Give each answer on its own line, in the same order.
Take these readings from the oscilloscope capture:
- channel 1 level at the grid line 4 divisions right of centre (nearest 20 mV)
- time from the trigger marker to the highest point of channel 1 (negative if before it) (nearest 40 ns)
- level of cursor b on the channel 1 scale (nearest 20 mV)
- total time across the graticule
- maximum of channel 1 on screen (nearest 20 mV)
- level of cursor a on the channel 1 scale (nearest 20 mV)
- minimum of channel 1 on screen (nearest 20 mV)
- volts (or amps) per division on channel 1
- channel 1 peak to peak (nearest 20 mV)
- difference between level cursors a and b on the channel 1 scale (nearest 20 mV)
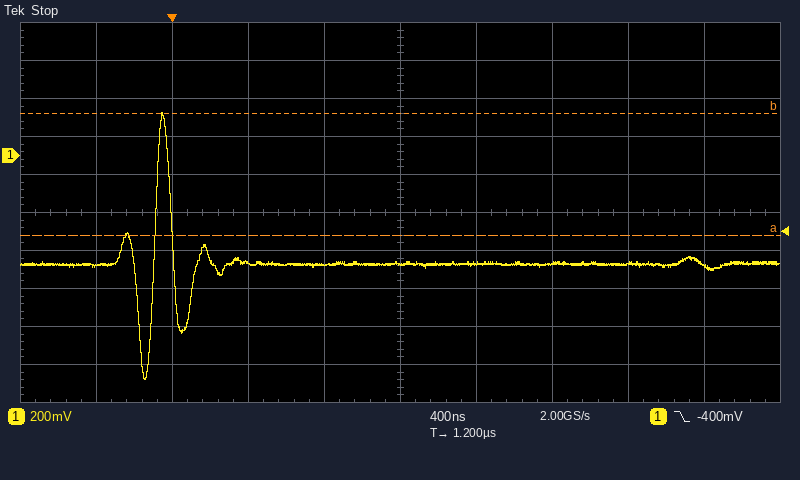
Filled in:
-580 mV
-40 ns
220 mV
4 µs
220 mV
-420 mV
-1.18 V
200 mV
1.40 V
640 mV
